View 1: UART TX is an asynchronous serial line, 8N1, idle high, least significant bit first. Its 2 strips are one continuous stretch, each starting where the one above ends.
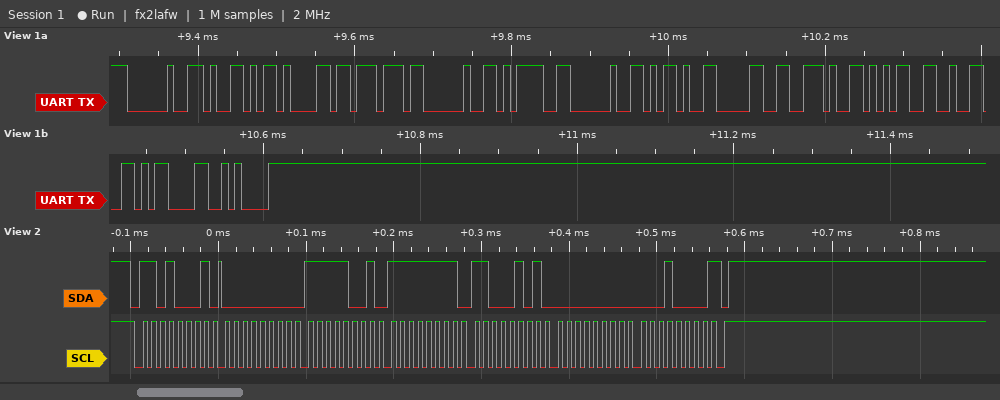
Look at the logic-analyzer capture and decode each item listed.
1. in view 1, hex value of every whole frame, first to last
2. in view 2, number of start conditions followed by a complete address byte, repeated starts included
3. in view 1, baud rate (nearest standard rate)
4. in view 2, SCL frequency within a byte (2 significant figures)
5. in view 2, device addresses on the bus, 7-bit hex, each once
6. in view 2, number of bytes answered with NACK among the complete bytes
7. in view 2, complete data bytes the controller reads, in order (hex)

0x20 0x59 0x61 0x77 0x20 0x3D 0x20 0x2D 0x30 0x2E 0x35 0x32 0x0D 0x0A
1
115200 baud
100 kHz
0x68
1
00 F9 FF C5 00 10
